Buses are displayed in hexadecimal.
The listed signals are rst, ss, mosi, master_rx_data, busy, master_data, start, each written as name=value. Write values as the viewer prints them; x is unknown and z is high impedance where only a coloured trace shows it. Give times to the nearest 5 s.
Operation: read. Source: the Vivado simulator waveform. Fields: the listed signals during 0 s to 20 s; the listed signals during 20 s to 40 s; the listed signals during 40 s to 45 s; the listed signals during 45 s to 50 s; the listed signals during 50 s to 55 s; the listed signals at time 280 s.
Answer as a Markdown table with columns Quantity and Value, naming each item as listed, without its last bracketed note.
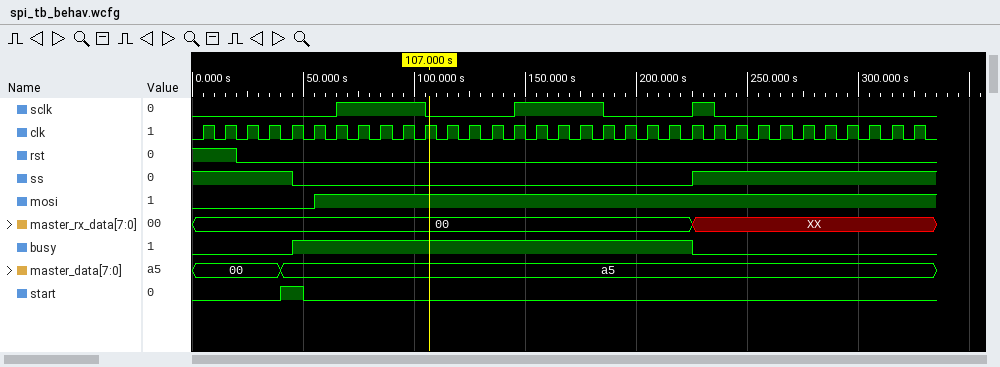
| Quantity | Value |
|---|---|
| the listed signals during 0 s to 20 s | rst=1, ss=1, mosi=0, master_rx_data=00, busy=0, master_data=00, start=0 |
| the listed signals during 20 s to 40 s | rst=0, ss=1, mosi=0, master_rx_data=00, busy=0, master_data=00, start=0 |
| the listed signals during 40 s to 45 s | rst=0, ss=1, mosi=0, master_rx_data=00, busy=0, master_data=a5, start=1 |
| the listed signals during 45 s to 50 s | rst=0, ss=0, mosi=0, master_rx_data=00, busy=1, master_data=a5, start=1 |
| the listed signals during 50 s to 55 s | rst=0, ss=0, mosi=0, master_rx_data=00, busy=1, master_data=a5, start=0 |
| the listed signals at time 280 s | rst=0, ss=1, mosi=1, master_rx_data=XX, busy=0, master_data=a5, start=0 |
